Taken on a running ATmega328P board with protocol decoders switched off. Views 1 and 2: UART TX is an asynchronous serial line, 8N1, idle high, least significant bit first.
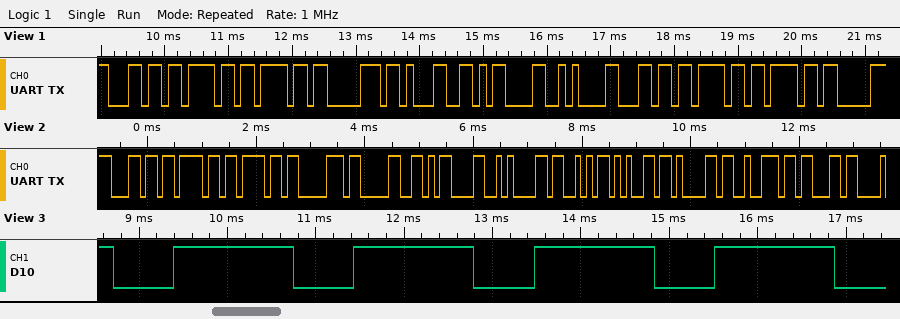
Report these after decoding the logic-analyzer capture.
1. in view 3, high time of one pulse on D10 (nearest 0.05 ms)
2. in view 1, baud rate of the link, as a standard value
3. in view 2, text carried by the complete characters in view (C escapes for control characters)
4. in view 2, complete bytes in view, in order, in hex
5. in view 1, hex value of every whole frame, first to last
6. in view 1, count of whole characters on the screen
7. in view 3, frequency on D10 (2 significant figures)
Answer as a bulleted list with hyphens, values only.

- 1.35 ms
- 9600 baud
- "loop0\r\nSearc"
- 6C 6F 6F 70 30 0D 0A 53 65 61 72 63
- 0x6C 0x6F 0x6F 0x70 0x31 0x0D 0x0A 0x6C 0x6F 0x6F
- 10
- 490 Hz
